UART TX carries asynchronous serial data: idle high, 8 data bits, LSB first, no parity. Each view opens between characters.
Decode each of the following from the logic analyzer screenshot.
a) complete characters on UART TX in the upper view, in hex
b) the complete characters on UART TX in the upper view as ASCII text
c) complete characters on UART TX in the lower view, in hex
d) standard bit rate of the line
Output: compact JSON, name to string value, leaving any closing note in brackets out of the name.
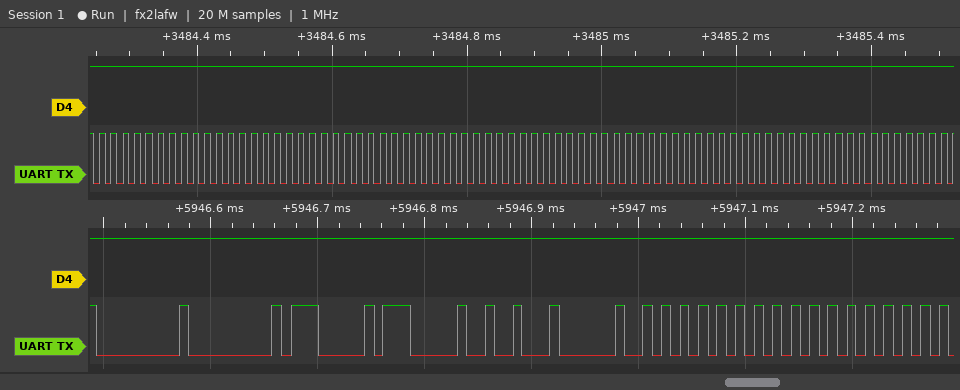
{"complete characters on UART TX in the upper view, in hex": "55, 55, 55, 55, 55, 55, 55, 55, 55, 55, 55, 55, 55, 55", "the complete characters on UART TX in the upper view as ASCII text": "\"UUUUUUUUUUUUUU\"", "complete characters on UART TX in the lower view, in hex": "00, 00, 07, 07, 12, 20, 55, 55, 55", "standard bit rate of the line": "115200 baud"}
